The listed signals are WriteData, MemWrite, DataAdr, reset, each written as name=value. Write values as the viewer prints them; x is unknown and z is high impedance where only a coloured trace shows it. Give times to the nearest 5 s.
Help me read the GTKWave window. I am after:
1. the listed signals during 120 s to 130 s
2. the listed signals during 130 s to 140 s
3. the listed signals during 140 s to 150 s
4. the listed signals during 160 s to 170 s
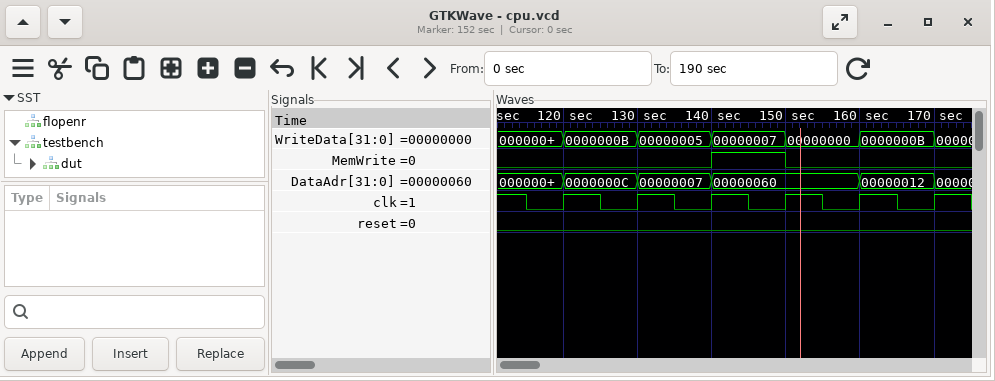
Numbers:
WriteData=0000000B, MemWrite=0, DataAdr=0000000C, reset=0
WriteData=00000005, MemWrite=0, DataAdr=00000007, reset=0
WriteData=00000007, MemWrite=1, DataAdr=00000060, reset=0
WriteData=0000000B, MemWrite=0, DataAdr=00000012, reset=0
